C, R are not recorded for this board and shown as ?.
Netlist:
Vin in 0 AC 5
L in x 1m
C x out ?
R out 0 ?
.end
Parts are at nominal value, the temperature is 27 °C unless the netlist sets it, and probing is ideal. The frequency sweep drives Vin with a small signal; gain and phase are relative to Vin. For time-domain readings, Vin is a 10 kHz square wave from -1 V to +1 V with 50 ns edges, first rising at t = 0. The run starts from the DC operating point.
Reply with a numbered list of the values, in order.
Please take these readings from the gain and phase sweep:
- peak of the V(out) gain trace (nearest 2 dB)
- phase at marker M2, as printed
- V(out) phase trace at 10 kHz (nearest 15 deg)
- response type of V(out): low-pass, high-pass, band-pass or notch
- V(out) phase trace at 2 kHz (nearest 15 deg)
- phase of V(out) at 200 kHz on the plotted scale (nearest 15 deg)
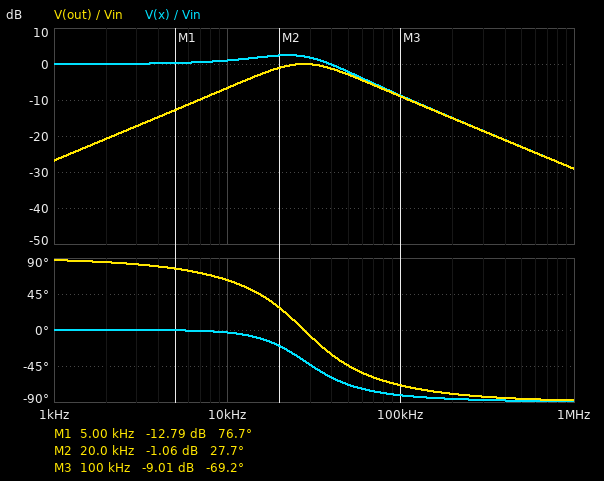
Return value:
1. 0 dB
2. 27.7 deg
3. 60 deg
4. band-pass
5. 90 deg
6. -75 deg
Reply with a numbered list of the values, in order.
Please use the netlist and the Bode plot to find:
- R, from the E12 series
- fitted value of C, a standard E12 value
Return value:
1. 220 Ω
2. 33 nF
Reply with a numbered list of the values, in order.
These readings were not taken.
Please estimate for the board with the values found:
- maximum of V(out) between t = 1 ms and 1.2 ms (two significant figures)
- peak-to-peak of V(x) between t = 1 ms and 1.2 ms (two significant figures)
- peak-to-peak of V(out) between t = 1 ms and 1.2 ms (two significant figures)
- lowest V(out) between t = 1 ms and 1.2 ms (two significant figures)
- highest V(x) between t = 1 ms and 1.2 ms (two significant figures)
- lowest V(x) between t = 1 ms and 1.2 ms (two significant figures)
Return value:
1. 1.2 V
2. 2.9 V
3. 2.4 V
4. -1.2 V
5. 1.5 V
6. -1.5 V
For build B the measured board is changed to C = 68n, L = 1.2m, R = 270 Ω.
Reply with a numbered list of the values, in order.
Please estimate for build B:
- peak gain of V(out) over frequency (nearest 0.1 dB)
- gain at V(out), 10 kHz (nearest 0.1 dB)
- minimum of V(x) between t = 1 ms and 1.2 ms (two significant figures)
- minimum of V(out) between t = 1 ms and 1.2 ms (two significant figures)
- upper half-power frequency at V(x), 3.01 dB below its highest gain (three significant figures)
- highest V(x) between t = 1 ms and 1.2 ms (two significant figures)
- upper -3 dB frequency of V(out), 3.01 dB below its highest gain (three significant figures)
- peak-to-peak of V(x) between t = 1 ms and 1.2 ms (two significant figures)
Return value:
1. 0 dB
2. -1.3 dB
3. -1.3 V
4. -1.4 V
5. 36.2 kHz
6. 1.3 V
7. 43.0 kHz
8. 2.5 V
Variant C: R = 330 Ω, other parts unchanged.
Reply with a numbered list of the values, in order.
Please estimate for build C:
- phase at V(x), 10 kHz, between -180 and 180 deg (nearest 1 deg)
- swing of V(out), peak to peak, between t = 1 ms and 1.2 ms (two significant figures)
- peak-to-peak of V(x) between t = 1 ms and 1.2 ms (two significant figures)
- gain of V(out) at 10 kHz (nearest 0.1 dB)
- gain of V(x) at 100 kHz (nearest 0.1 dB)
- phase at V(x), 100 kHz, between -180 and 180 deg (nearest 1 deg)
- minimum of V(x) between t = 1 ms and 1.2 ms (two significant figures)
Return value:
1. -4 deg
2. 2.9 V
3. 2.6 V
4. -4.2 dB
5. -6.0 dB
6. -69 deg
7. -1.3 V
